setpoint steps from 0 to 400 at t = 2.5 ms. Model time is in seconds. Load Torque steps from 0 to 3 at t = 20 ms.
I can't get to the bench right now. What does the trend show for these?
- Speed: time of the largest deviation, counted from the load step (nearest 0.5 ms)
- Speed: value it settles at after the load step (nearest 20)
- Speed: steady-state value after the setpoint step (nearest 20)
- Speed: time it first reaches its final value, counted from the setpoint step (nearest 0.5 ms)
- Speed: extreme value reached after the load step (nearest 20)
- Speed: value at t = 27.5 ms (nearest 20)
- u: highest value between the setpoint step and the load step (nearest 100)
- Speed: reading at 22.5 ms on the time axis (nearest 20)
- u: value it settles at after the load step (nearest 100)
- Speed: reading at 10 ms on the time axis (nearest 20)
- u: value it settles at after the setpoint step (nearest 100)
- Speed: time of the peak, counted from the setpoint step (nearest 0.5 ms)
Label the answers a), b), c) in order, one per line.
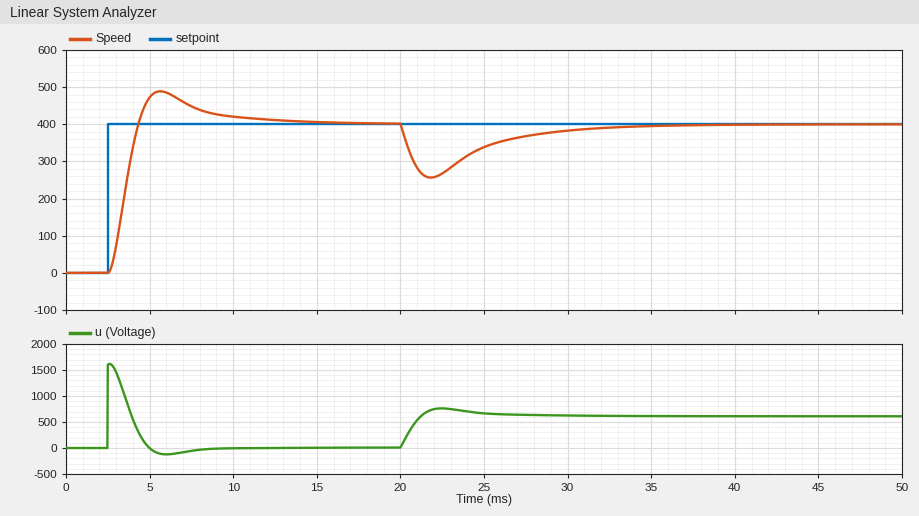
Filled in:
a) 2.0 ms
b) 400
c) 400
d) 2.0 ms
e) 260
f) 360
g) 1600
h) 260
i) 600
j) 420
k) 0
l) 3.0 ms
